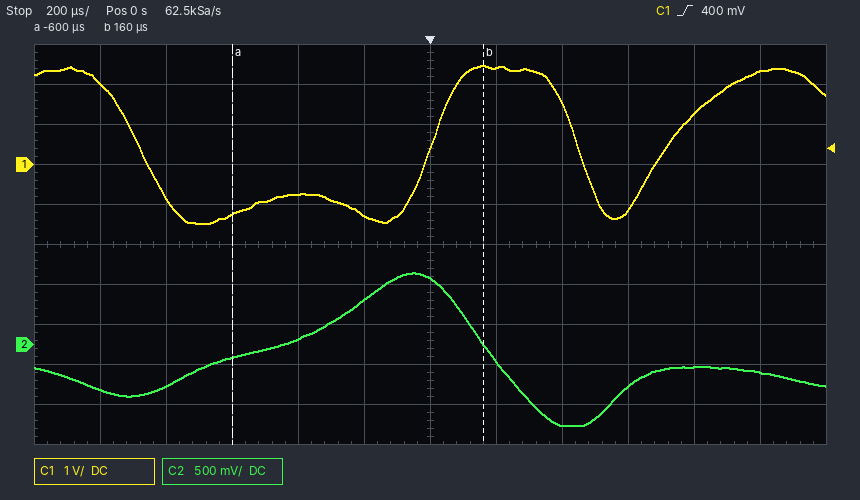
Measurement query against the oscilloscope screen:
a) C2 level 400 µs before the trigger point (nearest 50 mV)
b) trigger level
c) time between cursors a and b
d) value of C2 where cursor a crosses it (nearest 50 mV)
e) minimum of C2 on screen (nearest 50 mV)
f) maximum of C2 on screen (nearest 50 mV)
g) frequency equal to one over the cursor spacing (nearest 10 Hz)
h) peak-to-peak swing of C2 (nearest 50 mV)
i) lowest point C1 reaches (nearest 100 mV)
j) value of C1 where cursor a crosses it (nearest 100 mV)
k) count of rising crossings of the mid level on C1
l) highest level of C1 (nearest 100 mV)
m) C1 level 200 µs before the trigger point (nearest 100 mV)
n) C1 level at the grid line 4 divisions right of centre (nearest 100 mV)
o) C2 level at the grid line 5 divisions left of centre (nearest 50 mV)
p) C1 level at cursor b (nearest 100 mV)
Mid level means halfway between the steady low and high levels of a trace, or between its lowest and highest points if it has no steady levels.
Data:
50 mV
400 mV
760 µs
-150 mV
-1.00 V
900 mV
1.32 kHz
1.90 V
-1.5 V
-1.2 V
2
2.5 V
-1.3 V
1.3 V
-550 mV
2.5 V
